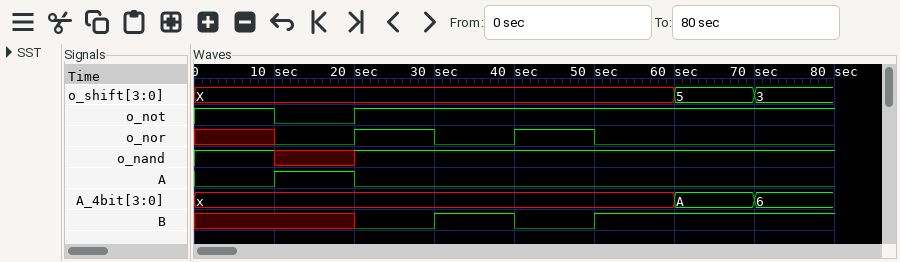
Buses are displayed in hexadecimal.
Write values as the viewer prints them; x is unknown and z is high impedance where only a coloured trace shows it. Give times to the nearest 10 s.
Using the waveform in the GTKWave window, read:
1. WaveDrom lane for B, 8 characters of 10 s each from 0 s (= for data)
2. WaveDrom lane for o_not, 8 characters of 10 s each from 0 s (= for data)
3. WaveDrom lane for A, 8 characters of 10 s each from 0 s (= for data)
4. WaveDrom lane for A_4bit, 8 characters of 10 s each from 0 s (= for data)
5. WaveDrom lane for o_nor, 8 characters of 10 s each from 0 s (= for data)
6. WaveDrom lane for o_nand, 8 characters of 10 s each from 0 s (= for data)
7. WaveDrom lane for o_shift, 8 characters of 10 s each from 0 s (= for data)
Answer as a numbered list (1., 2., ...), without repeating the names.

1. {name: 'B', wave: 'x.0101..'}
2. {name: 'o_not', wave: '101.....'}
3. {name: 'A', wave: '010.....'}
4. {name: 'A_4bit', wave: 'x.....==', data: 'A 6'}
5. {name: 'o_nor', wave: 'x01010..'}
6. {name: 'o_nand', wave: '1x1.....'}
7. {name: 'o_shift', wave: '=.....==', data: 'X 5 3'}
